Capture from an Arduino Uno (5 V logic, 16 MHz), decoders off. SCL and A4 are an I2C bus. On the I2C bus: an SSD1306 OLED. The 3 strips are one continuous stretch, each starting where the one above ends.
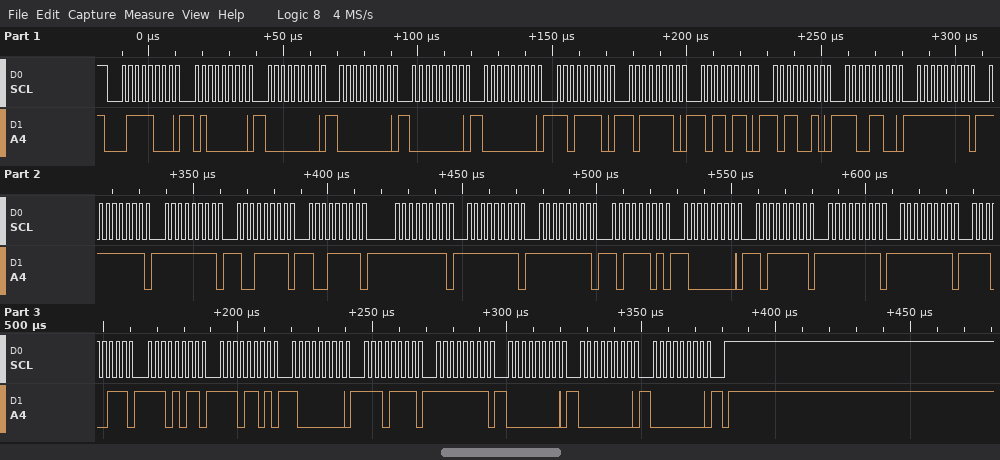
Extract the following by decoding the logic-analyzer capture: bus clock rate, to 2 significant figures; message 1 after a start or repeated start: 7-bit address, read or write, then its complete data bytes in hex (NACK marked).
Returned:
400 kHz
0x3C write: 40 00 00 00 00 DE BE B6 B2 CC FF FF FF 9F 9F FF FF FF BD 80 BF FF FF E7 EB ED 80 EF FF 00 00 00
